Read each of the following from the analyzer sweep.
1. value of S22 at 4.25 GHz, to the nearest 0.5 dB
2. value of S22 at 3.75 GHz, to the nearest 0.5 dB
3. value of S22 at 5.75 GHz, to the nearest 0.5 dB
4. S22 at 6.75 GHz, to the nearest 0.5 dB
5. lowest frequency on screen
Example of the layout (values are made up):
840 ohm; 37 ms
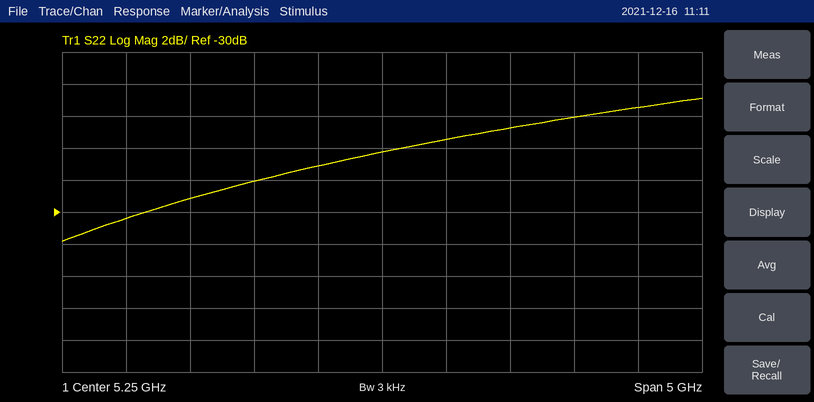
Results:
-28.0 dB; -29.0 dB; -25.5 dB; -24.0 dB; 2.75 GHz
